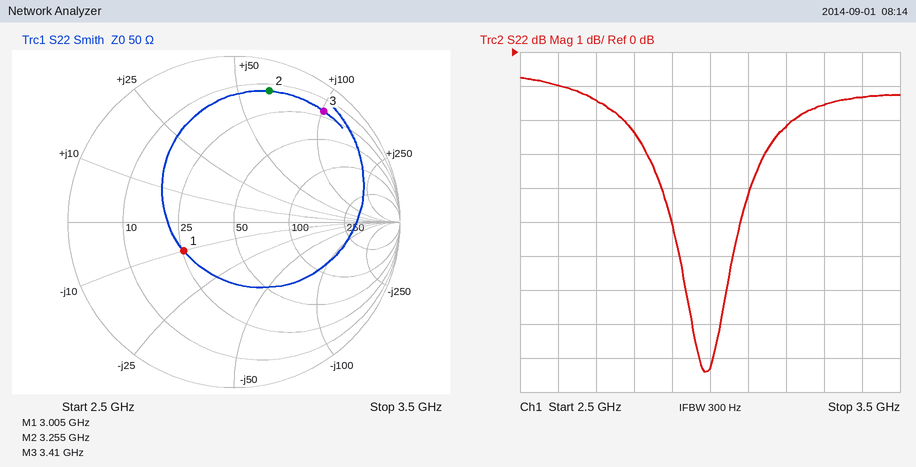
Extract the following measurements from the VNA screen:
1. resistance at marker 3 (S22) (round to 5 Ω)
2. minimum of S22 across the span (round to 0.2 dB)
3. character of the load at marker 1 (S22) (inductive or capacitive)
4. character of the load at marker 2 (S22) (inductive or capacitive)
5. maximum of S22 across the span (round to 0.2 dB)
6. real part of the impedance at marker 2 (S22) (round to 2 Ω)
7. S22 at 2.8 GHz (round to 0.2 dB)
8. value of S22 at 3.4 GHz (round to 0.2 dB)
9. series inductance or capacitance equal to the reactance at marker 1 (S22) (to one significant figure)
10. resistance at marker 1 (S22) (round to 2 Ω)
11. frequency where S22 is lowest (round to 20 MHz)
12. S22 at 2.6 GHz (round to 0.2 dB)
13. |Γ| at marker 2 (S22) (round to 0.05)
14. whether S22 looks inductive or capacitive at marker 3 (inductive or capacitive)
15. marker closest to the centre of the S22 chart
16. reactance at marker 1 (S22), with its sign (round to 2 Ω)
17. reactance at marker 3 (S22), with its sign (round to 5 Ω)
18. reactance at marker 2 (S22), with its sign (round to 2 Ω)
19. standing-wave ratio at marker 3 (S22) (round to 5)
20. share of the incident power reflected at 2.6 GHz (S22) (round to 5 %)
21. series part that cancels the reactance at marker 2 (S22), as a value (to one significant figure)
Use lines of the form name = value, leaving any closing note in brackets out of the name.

resistance at marker 3 (S22) = 20 Ω
minimum of S22 across the span = -9.4 dB
character of the load at marker 1 (S22) = capacitive
character of the load at marker 2 (S22) = inductive
maximum of S22 across the span = -0.8 dB
real part of the impedance at marker 2 (S22) = 14 Ω
S22 at 2.8 GHz = -2.4 dB
value of S22 at 3.4 GHz = -1.4 dB
series inductance or capacitance equal to the reactance at marker 1 (S22) = 5 pF
resistance at marker 1 (S22) = 26 Ω
frequency where S22 is lowest = 2.98 GHz
S22 at 2.6 GHz = -1.0 dB
|Γ| at marker 2 (S22) = 0.80
whether S22 looks inductive or capacitive at marker 3 = inductive
marker closest to the centre of the S22 chart = marker 1
reactance at marker 1 (S22), with its sign = -10 Ω
reactance at marker 3 (S22), with its sign = +100 Ω
reactance at marker 2 (S22), with its sign = +64 Ω
standing-wave ratio at marker 3 (S22) = 15
share of the incident power reflected at 2.6 GHz (S22) = 80 %
series part that cancels the reactance at marker 2 (S22), as a value = 800 fF
